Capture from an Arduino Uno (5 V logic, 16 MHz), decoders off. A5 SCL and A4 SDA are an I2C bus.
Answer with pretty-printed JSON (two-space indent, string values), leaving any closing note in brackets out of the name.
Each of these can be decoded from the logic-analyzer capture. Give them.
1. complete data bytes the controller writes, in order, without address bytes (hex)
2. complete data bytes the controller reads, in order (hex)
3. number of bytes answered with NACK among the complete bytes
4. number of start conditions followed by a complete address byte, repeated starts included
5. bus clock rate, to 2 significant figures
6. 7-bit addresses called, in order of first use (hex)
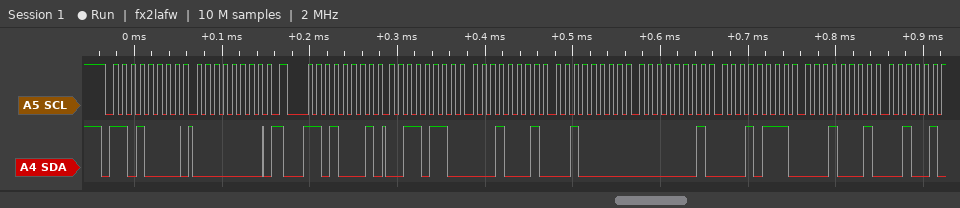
{
  "complete data bytes the controller writes, in order, without address bytes": "00",
  "complete data bytes the controller reads, in order": "36 11 20 01 17 11",
  "number of bytes answered with NACK among the complete bytes": "0",
  "number of start conditions followed by a complete address byte, repeated starts included": "2",
  "bus clock rate, to 2 significant figures": "100 kHz",
  "7-bit addresses called, in order of first use": "0x68"
}
